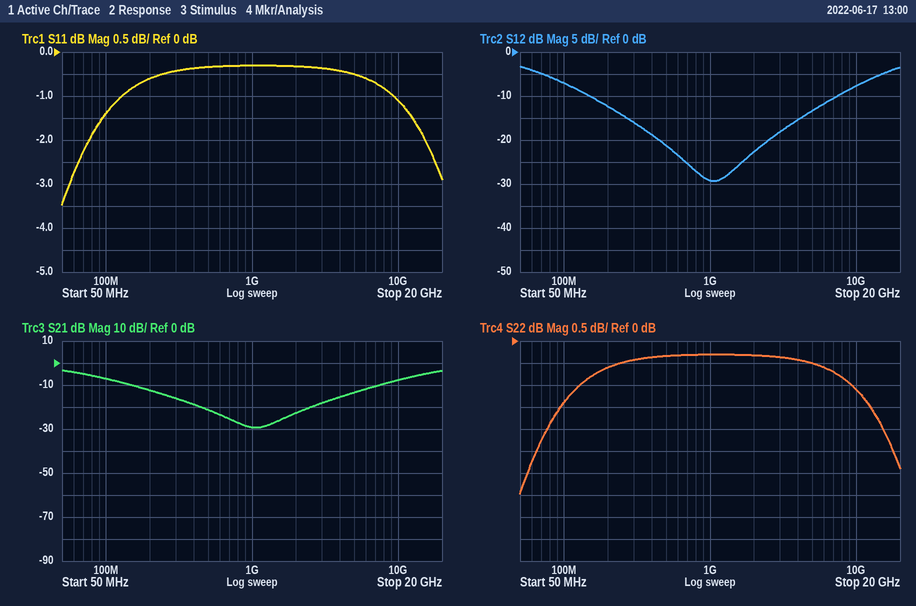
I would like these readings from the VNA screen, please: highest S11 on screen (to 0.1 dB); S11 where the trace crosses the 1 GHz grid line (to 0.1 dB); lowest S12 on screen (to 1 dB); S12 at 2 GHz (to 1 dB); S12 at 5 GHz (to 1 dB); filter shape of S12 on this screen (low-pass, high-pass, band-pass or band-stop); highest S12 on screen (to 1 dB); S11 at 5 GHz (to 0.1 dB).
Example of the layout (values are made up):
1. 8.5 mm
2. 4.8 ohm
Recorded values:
1. -0.3 dB
2. -0.3 dB
3. -29 dB
4. -23 dB
5. -13 dB
6. band-stop
7. -3 dB
8. -0.5 dB
